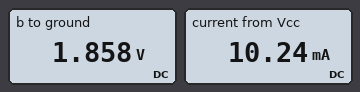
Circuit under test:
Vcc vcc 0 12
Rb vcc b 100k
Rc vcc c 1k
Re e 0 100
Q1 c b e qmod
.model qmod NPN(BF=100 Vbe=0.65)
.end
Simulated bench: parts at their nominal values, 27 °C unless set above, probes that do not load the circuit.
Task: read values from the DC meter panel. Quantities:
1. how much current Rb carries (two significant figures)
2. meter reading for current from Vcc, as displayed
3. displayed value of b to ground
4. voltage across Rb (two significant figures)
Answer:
100 µA
10.24 mA
1.858 V
10 V
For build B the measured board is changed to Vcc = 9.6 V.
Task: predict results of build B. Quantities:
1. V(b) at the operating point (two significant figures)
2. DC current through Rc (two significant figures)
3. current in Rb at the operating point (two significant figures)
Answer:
1.6 V
8.0 mA
80 µA
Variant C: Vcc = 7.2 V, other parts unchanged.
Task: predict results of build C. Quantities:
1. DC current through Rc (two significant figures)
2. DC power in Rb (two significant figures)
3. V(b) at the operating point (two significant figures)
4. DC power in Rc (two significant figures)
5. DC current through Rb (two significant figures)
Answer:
5.8 mA
340 µW
1.4 V
34 mW
58 µA
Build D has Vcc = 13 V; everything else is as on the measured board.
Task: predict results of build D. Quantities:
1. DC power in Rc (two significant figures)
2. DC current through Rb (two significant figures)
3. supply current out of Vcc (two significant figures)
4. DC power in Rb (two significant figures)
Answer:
120 mW
110 µA
11 mA
1.2 mW
